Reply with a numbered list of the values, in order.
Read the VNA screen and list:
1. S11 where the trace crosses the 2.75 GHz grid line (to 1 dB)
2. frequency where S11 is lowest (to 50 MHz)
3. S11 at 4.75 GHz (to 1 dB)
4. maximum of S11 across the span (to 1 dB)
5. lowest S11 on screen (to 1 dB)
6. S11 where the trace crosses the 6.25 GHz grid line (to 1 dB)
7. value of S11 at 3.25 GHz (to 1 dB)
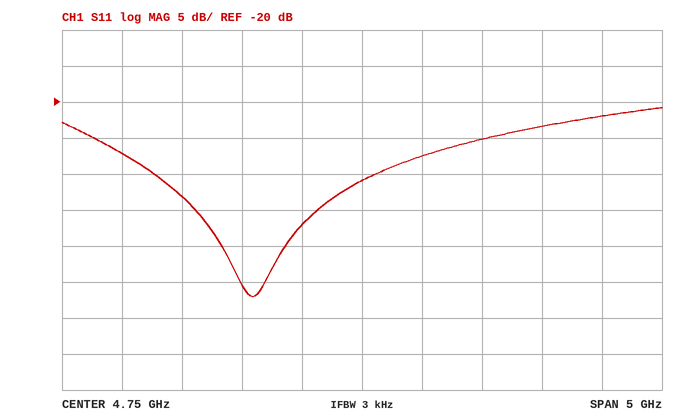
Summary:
1. -27 dB
2. 3.85 GHz
3. -31 dB
4. -21 dB
5. -47 dB
6. -23 dB
7. -33 dB
